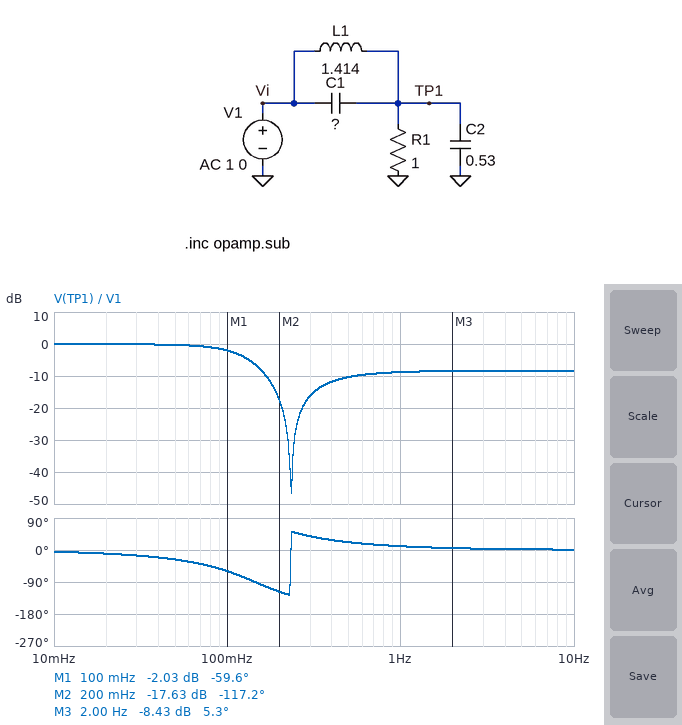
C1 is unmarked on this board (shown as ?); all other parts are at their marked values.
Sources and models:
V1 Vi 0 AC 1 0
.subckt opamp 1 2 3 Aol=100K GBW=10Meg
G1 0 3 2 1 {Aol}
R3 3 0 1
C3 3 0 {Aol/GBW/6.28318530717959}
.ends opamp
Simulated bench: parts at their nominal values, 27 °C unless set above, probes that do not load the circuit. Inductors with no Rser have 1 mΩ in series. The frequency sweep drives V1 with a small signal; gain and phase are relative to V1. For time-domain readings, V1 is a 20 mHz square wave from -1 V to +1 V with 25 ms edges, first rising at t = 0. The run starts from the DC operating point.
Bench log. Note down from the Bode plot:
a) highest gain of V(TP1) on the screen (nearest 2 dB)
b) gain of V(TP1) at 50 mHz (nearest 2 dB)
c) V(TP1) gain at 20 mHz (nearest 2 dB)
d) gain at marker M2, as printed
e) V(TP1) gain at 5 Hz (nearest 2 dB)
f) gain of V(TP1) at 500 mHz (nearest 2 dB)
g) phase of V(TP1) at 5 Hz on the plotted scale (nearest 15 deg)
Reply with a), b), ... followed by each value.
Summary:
a) 0 dB
b) 0 dB
c) 0 dB
d) -17.63 dB
e) -8 dB
f) -10 dB
g) 0 deg
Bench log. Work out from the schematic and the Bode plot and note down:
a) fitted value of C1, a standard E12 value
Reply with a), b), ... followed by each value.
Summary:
a) 330 mF
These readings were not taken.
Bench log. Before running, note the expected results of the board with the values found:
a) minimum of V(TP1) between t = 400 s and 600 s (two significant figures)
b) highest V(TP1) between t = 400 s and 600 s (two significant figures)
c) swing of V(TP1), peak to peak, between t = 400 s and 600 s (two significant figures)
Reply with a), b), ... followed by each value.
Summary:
a) -1.1 V
b) 1.1 V
c) 2.2 V
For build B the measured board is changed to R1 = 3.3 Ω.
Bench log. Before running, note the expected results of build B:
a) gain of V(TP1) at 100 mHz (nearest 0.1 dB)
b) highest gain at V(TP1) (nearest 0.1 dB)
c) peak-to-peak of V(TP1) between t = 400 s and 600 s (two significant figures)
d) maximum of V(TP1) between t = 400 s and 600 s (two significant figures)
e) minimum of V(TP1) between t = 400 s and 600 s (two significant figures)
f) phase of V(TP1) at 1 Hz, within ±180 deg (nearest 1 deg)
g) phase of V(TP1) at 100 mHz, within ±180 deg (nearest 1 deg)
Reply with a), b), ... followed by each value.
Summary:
a) 2.9 dB
b) 4.8 dB
c) 3.4 V
d) 1.7 V
e) -1.7 V
f) 3 deg
g) -27 deg
